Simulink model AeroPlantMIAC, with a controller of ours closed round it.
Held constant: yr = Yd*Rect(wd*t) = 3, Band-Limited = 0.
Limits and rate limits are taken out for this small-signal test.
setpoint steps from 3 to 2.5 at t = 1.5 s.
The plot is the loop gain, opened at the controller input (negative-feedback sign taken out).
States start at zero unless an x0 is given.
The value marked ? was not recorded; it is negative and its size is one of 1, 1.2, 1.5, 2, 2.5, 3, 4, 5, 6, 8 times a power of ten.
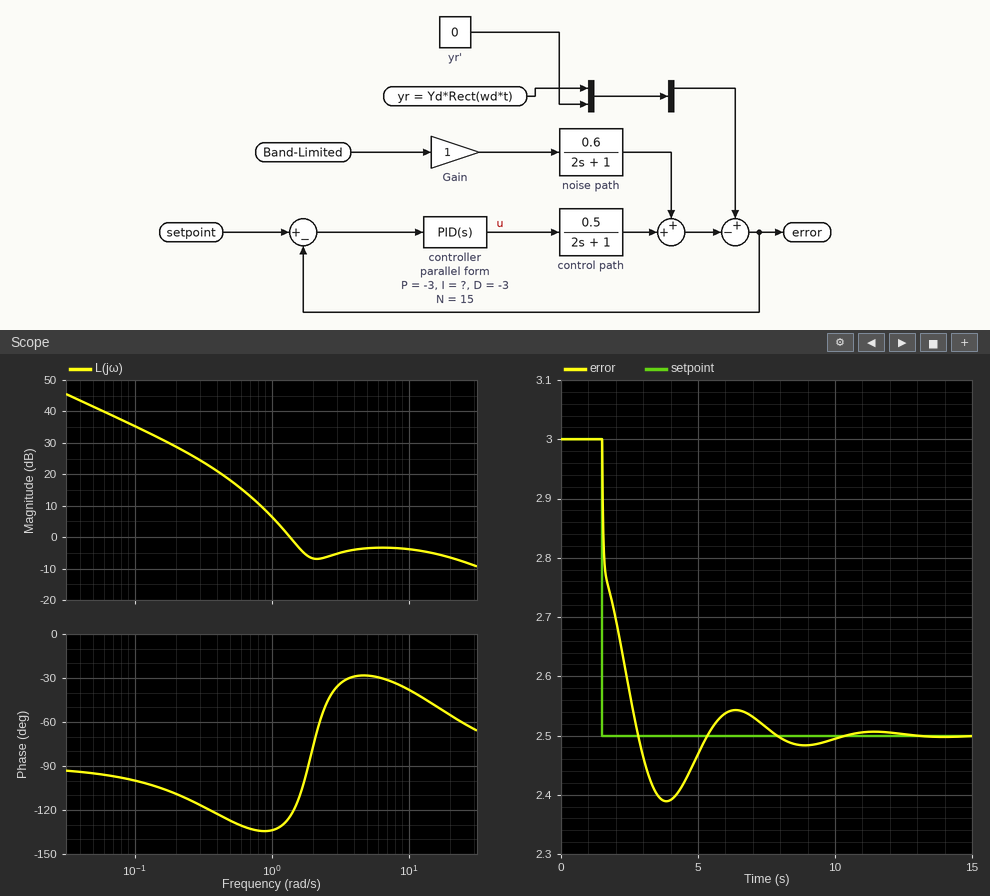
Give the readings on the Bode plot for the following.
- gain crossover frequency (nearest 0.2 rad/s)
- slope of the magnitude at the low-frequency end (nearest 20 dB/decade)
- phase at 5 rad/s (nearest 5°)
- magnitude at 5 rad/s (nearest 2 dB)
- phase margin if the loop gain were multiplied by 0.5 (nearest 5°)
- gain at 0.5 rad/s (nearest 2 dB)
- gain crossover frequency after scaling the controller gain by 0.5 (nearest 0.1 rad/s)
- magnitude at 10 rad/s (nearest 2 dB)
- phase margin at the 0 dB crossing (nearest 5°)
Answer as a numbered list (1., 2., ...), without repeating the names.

1. 1.4 rad/s
2. -20 dB/decade
3. -30°
4. -4 dB
5. 45°
6. 18 dB
7. 1.0 rad/s
8. -4 dB
9. 55°
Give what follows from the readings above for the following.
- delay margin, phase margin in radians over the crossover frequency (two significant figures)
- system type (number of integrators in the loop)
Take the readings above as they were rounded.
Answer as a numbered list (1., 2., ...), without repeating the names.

1. 0.69 s
2. 1
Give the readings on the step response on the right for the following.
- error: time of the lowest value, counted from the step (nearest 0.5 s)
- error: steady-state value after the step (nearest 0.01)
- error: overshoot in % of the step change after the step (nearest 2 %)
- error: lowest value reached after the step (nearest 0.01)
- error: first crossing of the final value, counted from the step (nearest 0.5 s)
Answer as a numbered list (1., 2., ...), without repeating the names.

1. 2.5 s
2. 2.50
3. 22 %
4. 2.39
5. 1.5 s
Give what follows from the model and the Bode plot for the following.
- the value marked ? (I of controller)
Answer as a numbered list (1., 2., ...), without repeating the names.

1. -12
